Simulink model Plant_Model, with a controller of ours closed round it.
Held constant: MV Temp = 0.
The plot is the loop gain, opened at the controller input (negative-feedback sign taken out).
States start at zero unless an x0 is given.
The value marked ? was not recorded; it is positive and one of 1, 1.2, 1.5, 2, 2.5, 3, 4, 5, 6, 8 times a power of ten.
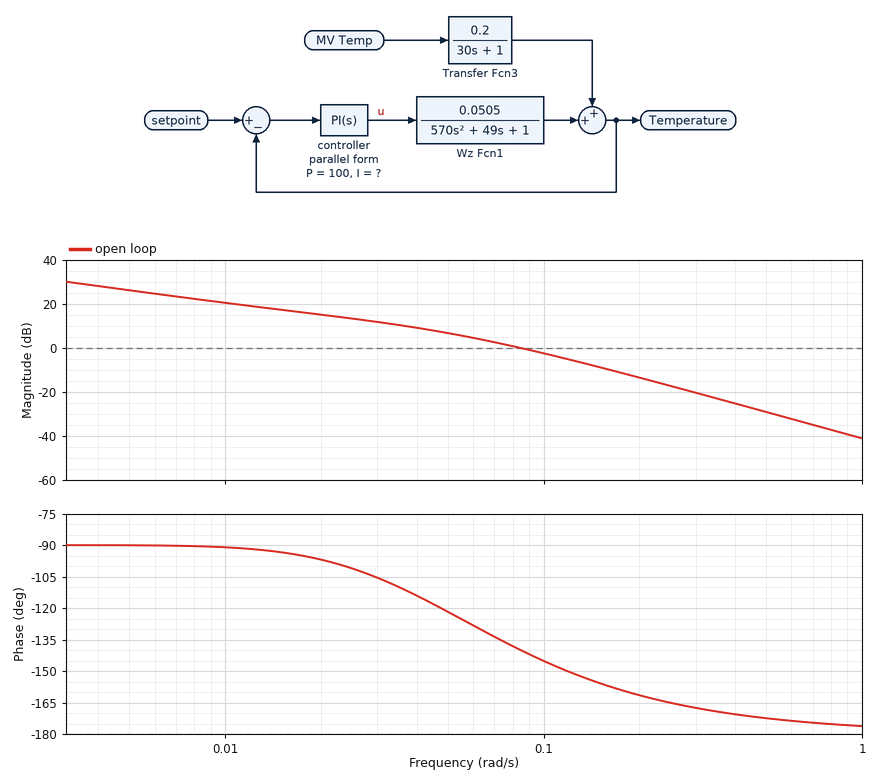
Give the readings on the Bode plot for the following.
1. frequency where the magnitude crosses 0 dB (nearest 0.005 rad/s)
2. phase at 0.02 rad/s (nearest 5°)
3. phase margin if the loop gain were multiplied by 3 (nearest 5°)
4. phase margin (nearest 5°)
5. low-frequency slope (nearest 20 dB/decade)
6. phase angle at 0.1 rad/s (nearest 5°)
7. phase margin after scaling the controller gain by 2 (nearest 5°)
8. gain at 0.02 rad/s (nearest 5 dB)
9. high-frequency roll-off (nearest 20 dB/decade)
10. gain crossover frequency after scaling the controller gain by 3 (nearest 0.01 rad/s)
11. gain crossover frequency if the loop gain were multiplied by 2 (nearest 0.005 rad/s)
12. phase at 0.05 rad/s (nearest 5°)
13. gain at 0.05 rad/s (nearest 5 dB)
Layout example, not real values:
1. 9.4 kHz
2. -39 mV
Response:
1. 0.085 rad/s
2. -95°
3. 25°
4. 40°
5. -20 dB/decade
6. -145°
7. 30°
8. 15 dB
9. -40 dB/decade
10. 0.16 rad/s
11. 0.125 rad/s
12. -120°
13. 5 dB
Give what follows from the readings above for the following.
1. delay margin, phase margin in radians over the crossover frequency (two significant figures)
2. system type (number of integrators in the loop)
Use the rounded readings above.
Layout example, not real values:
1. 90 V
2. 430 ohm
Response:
1. 8.2 s
2. 1
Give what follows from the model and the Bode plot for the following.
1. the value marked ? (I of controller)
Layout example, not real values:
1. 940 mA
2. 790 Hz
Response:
1. 2
